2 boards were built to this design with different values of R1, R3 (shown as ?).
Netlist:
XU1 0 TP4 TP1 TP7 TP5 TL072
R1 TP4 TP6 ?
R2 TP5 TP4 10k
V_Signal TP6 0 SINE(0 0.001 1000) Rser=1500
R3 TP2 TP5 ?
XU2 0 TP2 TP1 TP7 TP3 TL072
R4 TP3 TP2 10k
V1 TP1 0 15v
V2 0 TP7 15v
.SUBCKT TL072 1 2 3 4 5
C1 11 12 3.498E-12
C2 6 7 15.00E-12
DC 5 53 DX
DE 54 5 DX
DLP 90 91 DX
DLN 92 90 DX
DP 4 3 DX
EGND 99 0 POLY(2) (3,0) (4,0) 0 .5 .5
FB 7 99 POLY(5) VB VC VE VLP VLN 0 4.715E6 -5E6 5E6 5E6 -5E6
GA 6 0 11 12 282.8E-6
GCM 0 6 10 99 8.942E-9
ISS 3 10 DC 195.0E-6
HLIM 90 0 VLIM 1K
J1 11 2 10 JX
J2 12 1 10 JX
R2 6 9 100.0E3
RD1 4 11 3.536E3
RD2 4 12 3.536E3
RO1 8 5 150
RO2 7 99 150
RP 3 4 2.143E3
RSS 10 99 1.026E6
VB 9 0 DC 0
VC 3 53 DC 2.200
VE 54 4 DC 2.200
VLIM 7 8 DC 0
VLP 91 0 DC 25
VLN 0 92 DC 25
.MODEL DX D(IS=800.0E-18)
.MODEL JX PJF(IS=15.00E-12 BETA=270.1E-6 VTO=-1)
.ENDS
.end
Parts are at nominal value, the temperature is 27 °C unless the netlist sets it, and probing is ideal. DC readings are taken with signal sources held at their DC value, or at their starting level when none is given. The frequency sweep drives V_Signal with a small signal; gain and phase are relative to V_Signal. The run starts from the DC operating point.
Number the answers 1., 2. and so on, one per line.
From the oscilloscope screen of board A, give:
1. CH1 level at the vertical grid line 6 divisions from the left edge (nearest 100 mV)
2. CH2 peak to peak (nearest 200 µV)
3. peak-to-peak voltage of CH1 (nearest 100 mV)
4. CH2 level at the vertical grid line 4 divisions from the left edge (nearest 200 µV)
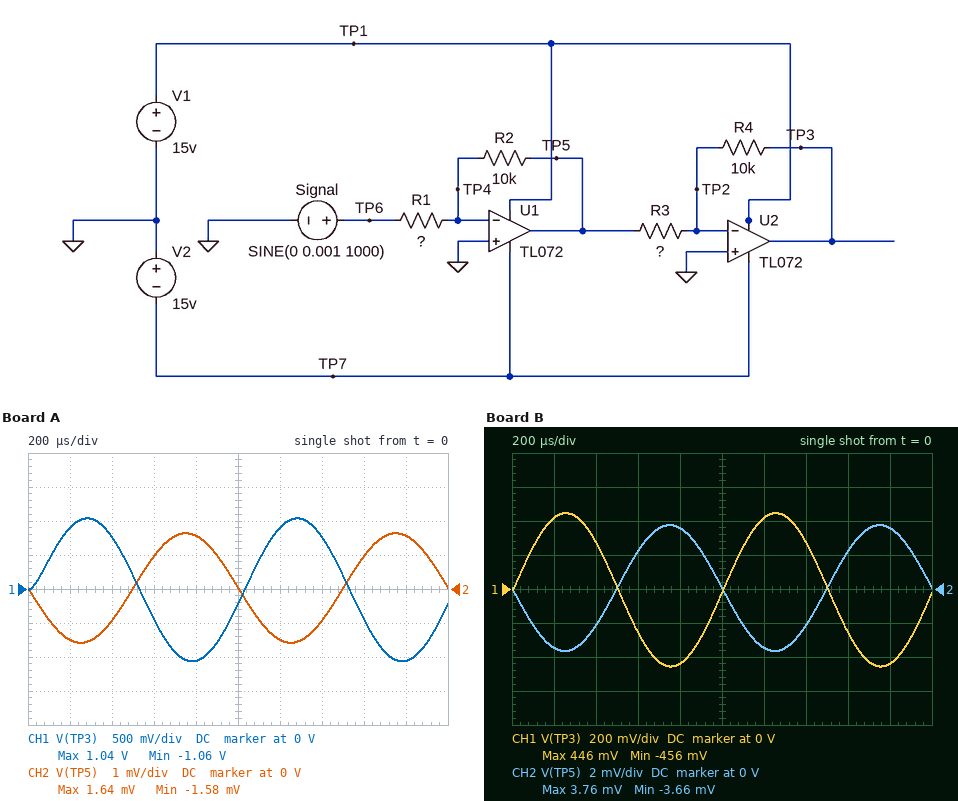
1. 900 mV
2. 3.2 mV
3. 2.1 V
4. 1.6 mV
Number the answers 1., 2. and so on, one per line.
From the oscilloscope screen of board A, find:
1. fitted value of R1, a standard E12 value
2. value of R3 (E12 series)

1. 4.7 kΩ
2. 15 Ω
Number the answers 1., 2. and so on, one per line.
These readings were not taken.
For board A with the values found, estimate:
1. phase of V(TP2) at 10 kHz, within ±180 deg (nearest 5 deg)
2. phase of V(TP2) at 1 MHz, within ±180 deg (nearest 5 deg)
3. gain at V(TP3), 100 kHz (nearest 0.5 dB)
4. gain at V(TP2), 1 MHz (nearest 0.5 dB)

1. -155 deg
2. 140 deg
3. 34.5 dB
4. 2.5 dB
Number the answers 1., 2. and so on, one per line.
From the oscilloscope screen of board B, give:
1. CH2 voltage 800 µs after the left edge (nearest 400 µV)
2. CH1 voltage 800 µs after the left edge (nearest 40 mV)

1. 3.6 mV
2. -440 mV
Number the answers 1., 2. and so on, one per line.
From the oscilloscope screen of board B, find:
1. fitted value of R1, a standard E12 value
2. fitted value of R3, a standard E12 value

1. 1.2 kΩ
2. 82 Ω
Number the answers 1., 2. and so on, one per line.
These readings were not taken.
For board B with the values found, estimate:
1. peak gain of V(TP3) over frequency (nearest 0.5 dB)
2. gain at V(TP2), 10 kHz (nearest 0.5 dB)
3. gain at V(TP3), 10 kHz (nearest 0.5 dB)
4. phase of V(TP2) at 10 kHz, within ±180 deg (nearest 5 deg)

1. 53.0 dB
2. 2.0 dB
3. 52.5 dB
4. -110 deg
